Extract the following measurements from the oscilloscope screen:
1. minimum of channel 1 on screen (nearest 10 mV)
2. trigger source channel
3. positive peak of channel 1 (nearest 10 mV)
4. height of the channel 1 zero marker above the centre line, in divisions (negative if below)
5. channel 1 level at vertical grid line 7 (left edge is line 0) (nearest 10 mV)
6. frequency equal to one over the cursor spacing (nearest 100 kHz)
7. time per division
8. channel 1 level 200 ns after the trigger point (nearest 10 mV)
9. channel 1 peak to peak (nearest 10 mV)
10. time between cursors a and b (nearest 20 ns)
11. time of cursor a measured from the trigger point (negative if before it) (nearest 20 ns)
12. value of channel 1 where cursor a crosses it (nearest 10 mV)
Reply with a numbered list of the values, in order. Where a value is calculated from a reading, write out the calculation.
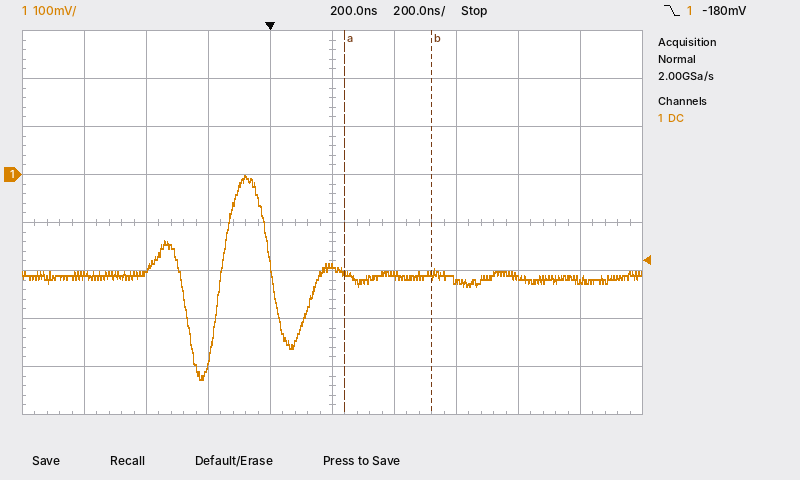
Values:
1. -430 mV
2. channel 1
3. 0 mV
4. +1.0 div
5. -220 mV
6. 1 / 280 ns ≈ 3.6 MHz
7. 200 ns
8. -190 mV
9. 0 mV − (-430 mV) = 430 mV
10. 280 ns
11. +240 ns
12. -200 mV
